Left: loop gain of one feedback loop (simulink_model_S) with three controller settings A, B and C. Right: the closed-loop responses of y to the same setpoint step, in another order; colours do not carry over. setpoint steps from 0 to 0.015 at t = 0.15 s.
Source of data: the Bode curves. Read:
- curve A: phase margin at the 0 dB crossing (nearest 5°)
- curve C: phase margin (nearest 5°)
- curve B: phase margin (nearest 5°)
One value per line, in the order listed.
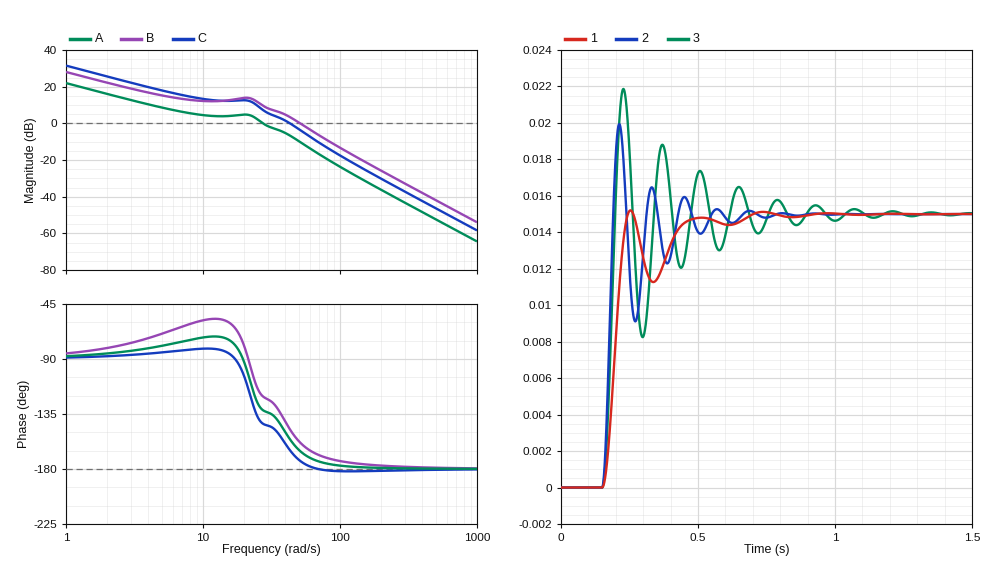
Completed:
50°
15°
20°
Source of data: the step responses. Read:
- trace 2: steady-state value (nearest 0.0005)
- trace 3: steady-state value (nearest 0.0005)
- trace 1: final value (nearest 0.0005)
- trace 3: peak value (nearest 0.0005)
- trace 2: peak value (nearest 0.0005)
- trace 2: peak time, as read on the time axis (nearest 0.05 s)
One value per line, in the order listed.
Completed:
0.0150
0.0150
0.0150
0.0220
0.0200
0.20 s
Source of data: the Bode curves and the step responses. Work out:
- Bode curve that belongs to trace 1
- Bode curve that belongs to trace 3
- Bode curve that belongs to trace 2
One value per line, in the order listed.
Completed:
A
C
B
